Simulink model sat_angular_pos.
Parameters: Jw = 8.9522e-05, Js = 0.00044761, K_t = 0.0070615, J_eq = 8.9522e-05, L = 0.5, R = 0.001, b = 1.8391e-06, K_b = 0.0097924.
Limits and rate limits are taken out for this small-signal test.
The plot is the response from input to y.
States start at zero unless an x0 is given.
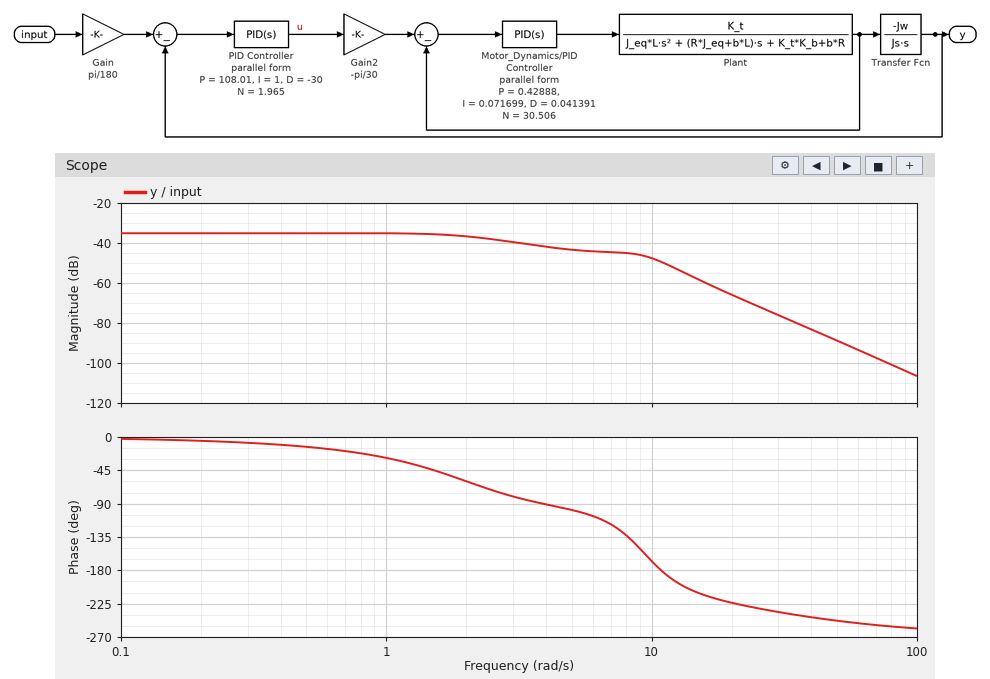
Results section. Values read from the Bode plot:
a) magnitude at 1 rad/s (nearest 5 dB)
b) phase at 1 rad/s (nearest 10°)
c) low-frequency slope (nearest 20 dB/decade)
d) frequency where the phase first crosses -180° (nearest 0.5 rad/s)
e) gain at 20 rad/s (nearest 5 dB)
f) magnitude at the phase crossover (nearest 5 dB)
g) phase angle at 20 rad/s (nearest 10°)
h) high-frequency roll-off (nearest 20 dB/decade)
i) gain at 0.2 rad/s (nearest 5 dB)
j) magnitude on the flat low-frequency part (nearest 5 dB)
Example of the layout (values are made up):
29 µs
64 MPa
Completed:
-35 dB
-30°
0 dB/decade
11.0 rad/s
-65 dB
-50 dB
-220°
-60 dB/decade
-35 dB
-35 dB
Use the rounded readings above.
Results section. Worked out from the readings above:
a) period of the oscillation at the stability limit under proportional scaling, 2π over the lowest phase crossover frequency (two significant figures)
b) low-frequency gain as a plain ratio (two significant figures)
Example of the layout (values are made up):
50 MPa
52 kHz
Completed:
0.57 s
0.018
